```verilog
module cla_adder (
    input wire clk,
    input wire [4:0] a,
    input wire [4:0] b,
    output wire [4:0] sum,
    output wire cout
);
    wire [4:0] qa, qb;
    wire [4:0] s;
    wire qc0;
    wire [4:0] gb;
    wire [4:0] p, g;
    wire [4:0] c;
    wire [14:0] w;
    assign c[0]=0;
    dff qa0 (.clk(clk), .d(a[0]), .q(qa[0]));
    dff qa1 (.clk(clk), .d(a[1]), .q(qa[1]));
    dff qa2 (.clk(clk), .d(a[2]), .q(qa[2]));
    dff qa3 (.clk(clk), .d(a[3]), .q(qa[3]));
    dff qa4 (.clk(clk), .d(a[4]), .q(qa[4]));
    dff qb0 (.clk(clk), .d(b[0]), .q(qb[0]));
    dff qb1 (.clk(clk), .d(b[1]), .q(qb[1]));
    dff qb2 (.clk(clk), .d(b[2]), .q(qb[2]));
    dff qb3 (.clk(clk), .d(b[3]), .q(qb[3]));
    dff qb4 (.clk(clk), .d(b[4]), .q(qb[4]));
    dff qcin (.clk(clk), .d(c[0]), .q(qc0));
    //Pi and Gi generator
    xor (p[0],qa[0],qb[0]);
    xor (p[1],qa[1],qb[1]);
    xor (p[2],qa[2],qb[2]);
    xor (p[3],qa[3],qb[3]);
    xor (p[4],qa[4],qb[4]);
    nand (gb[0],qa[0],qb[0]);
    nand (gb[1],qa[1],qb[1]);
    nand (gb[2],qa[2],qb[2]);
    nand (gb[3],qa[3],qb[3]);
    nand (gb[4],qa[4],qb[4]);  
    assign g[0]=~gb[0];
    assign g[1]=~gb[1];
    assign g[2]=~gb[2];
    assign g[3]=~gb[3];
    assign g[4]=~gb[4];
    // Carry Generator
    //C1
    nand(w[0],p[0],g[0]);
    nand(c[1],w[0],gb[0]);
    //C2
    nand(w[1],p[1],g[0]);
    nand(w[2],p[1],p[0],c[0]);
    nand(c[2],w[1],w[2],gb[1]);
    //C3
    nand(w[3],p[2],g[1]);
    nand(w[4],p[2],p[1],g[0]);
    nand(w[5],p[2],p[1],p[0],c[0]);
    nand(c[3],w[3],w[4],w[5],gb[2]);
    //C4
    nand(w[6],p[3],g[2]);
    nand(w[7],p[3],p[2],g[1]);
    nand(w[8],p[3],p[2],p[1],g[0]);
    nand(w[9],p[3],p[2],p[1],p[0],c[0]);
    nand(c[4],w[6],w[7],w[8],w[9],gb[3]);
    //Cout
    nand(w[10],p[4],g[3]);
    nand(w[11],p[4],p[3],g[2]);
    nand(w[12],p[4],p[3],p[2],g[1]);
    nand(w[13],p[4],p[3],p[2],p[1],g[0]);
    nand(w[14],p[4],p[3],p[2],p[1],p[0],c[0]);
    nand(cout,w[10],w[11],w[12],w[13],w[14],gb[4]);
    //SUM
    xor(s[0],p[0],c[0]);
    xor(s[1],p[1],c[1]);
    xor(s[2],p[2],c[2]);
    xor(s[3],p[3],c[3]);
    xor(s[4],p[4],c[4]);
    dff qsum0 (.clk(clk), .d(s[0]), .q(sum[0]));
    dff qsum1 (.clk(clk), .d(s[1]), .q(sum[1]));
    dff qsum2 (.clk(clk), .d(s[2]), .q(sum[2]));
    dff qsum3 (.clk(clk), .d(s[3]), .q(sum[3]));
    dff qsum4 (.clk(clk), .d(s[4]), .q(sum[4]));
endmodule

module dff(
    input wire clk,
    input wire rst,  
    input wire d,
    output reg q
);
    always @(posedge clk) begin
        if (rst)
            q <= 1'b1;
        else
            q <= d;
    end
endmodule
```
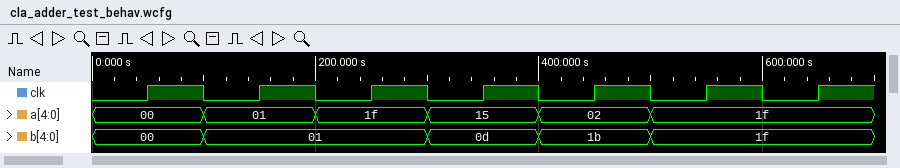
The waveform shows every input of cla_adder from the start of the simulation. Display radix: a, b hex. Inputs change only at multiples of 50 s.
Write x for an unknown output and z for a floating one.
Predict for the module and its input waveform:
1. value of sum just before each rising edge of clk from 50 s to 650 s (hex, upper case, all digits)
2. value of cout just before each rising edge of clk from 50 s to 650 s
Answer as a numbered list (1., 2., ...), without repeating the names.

1. x, x, 00, 02, 00, 02, 1D
2. x 0 0 1 1 0 1
